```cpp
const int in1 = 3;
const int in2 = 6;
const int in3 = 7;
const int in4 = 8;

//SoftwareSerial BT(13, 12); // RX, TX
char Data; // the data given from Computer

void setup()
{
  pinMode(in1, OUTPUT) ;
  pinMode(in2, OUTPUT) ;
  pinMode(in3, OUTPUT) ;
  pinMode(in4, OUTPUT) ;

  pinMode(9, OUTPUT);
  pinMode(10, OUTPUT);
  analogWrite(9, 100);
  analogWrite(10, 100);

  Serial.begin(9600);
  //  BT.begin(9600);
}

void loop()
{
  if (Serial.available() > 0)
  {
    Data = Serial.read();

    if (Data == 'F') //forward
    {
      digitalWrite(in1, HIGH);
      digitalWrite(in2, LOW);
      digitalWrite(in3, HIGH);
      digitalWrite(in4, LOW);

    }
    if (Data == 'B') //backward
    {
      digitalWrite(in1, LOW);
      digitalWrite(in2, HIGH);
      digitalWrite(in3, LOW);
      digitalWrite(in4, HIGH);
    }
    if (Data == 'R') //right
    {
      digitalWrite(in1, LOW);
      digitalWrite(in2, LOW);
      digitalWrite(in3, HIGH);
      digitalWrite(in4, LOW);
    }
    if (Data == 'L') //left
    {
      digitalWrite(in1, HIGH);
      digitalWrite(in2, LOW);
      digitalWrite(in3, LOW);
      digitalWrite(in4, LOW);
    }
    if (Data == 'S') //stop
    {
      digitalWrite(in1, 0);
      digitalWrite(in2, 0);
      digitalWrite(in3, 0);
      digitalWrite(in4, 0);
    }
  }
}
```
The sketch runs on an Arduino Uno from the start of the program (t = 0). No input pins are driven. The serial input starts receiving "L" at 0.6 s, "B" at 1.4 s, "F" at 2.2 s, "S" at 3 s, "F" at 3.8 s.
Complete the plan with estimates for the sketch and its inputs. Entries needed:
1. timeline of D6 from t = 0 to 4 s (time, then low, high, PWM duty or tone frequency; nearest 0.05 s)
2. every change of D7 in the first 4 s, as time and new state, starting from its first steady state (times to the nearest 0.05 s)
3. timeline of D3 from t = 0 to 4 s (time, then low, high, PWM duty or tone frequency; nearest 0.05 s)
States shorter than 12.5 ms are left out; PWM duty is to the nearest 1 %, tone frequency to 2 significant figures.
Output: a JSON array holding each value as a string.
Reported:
["0 s low; 1.4 s high; 2.2 s low", "0 s low; 2.2 s high; 3 s low; 3.8 s high", "0 s low; 0.6 s high; 1.4 s low; 2.2 s high; 3 s low; 3.8 s high"]
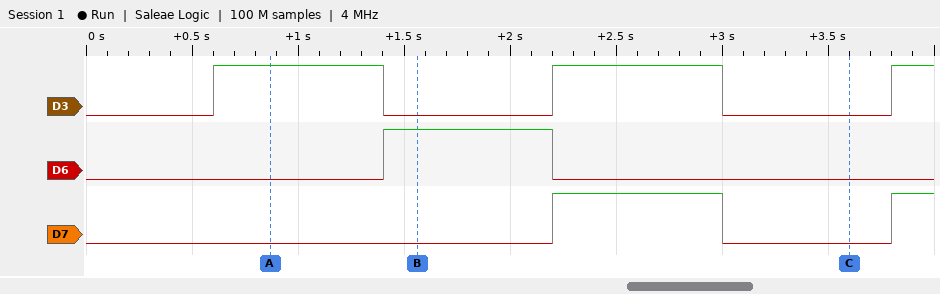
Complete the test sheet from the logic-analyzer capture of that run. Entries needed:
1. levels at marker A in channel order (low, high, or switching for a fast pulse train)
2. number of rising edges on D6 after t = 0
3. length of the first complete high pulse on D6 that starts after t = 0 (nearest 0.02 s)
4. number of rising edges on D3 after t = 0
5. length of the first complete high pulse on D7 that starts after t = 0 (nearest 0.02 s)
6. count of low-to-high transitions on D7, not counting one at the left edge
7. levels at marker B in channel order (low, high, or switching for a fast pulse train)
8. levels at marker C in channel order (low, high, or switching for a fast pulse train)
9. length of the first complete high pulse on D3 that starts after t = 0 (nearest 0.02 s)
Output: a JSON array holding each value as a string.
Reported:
["D3 high, D6 low, D7 low", "1", "0.80 s", "3", "0.80 s", "2", "D3 low, D6 high, D7 low", "D3 low, D6 low, D7 low", "0.80 s"]
